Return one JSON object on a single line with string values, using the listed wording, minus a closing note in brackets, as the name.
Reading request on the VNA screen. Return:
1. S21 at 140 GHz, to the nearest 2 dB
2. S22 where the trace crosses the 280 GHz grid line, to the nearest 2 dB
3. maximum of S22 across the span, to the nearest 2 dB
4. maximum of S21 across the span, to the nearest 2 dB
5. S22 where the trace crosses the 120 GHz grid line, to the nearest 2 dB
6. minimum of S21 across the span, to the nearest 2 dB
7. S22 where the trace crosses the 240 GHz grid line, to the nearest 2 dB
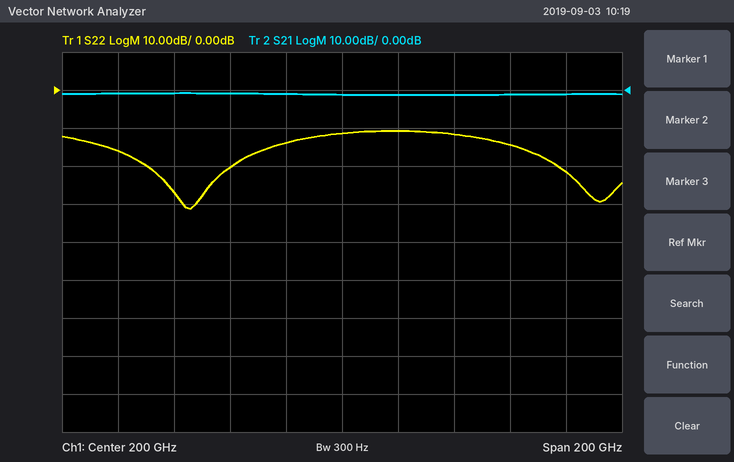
{"S21 at 140 GHz, to the nearest 2 dB": "0 dB", "S22 where the trace crosses the 280 GHz grid line, to the nearest 2 dB": "-22 dB", "maximum of S22 across the span, to the nearest 2 dB": "-10 dB", "maximum of S21 across the span, to the nearest 2 dB": "0 dB", "S22 where the trace crosses the 120 GHz grid line, to the nearest 2 dB": "-16 dB", "minimum of S21 across the span, to the nearest 2 dB": "-2 dB", "S22 where the trace crosses the 240 GHz grid line, to the nearest 2 dB": "-12 dB"}
